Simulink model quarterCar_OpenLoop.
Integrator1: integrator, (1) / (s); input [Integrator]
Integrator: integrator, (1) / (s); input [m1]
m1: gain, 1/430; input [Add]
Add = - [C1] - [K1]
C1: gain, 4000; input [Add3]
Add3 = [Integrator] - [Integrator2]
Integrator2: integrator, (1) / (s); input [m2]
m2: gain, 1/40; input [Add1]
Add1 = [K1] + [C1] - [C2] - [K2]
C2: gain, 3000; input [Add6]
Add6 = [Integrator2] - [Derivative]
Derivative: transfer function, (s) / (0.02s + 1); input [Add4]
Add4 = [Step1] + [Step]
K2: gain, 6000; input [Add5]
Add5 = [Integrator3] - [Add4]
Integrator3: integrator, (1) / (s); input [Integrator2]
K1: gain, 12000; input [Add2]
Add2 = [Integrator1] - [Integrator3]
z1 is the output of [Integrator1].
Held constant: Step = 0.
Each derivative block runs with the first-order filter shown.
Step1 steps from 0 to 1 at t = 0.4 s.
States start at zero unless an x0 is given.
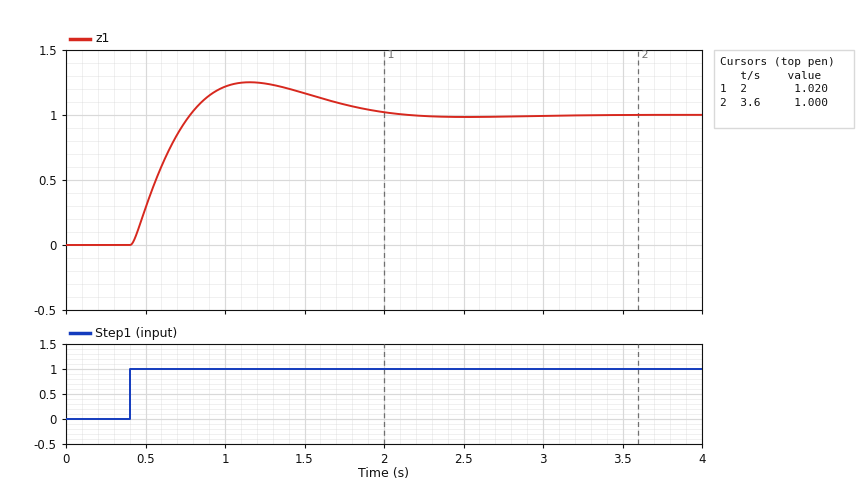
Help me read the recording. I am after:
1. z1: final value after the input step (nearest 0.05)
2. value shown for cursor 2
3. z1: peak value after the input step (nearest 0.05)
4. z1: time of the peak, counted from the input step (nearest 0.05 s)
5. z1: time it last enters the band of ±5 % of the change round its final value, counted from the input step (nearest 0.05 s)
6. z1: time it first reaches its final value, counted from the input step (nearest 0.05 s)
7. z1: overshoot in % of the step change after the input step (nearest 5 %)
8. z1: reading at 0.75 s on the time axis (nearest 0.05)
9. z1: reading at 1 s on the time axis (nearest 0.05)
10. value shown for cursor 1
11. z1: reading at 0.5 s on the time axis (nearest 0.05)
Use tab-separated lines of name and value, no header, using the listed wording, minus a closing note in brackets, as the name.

z1: final value after the input step	1.00
value shown for cursor 2	1.000
z1: peak value after the input step	1.25
z1: time of the peak, counted from the input step	0.75 s
z1: time it last enters the band of ±5 % of the change round its final value, counted from the input step	1.45 s
z1: time it first reaches its final value, counted from the input step	0.40 s
z1: overshoot in % of the step change after the input step	25 %
z1: reading at 0.75 s on the time axis	0.95
z1: reading at 1 s on the time axis	1.20
value shown for cursor 1	1.020
z1: reading at 0.5 s on the time axis	0.30
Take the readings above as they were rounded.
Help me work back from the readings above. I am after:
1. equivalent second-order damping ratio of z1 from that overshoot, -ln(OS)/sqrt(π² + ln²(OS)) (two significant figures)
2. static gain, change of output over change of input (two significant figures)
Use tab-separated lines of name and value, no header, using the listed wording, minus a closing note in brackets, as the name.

equivalent second-order damping ratio of z1 from that overshoot, -ln(OS)/sqrt(π² + ln²(OS))	0.40
static gain, change of output over change of input	1.0
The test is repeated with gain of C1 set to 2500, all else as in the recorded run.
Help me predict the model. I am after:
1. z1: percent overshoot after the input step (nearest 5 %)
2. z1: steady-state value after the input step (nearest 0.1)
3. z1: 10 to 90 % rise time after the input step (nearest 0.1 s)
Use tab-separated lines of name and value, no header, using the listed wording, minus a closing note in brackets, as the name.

z1: percent overshoot after the input step	30 %
z1: steady-state value after the input step	1.0
z1: 10 to 90 % rise time after the input step	0.3 s
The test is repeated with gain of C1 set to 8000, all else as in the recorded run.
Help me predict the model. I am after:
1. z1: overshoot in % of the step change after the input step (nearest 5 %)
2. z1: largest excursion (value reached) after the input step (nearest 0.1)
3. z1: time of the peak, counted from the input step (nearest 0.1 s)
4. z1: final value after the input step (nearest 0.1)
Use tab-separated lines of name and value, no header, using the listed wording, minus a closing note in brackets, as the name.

z1: overshoot in % of the step change after the input step	20 %
z1: largest excursion (value reached) after the input step	1.2
z1: time of the peak, counted from the input step	0.7 s
z1: final value after the input step	1.0
